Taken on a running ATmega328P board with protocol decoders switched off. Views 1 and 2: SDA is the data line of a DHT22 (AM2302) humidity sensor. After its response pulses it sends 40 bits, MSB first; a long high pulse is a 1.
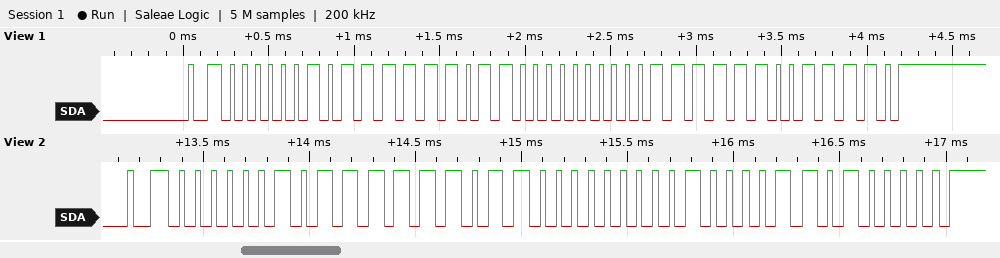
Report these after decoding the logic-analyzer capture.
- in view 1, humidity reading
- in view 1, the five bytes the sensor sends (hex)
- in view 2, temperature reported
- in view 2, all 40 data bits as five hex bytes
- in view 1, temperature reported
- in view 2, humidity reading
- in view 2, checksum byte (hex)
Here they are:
76.5 %
02 FD 80 1F 9E
-3.3 °C
02 FD 80 21 A0
-3.1 °C
76.5 %
0xA0
